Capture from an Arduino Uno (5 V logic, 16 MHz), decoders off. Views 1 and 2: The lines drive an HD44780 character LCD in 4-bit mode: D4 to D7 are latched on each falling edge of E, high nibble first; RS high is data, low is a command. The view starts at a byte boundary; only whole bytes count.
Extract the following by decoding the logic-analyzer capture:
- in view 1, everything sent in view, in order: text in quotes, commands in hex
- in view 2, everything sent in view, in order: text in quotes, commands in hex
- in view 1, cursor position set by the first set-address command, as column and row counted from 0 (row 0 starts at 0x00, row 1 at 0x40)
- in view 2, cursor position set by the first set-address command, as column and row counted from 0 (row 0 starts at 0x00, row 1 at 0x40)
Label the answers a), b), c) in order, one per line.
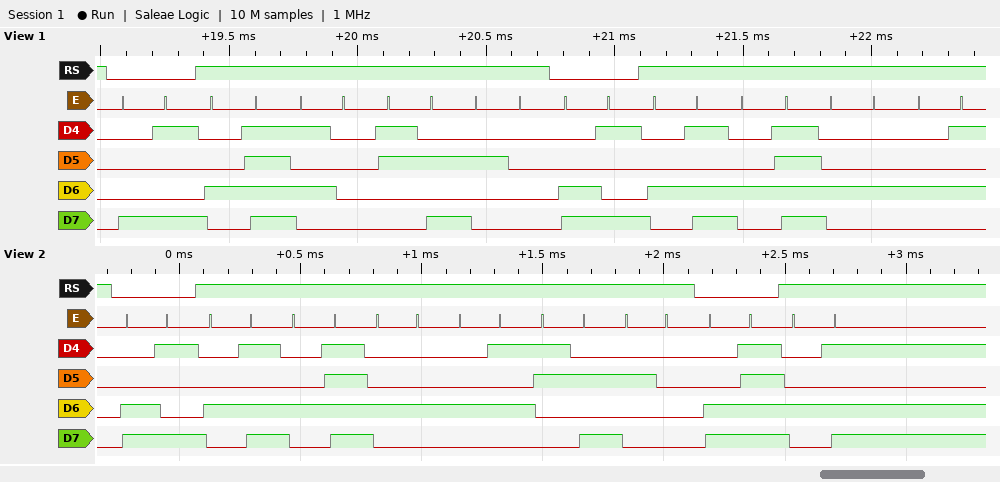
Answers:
a) 0x89 "OP: " 0xC9 "MODE"
b) 0xC9 "MODE: " 0xCF "M"
c) column 9, row 0
d) column 9, row 1
